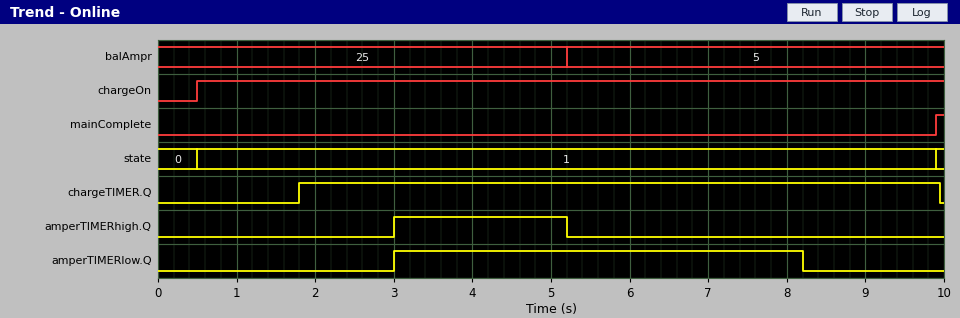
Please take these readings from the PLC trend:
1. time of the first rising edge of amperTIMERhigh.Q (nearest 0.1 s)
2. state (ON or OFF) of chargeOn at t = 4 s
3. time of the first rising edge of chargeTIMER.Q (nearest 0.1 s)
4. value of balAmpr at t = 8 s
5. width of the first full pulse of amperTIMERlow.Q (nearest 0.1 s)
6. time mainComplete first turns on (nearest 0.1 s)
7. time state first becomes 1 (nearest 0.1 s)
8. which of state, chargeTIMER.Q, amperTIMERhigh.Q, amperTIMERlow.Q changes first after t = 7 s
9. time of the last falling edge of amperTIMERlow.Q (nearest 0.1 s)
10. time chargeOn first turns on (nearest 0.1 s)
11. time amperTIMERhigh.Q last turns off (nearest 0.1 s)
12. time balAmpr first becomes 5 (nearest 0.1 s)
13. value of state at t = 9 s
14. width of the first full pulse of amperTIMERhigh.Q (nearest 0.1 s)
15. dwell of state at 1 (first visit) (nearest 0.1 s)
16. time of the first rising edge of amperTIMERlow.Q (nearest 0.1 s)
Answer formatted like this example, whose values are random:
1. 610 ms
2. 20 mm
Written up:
1. 3.0 s
2. ON
3. 1.8 s
4. 5
5. 5.2 s
6. 9.9 s
7. 0.5 s
8. amperTIMERlow.Q
9. 8.2 s
10. 0.5 s
11. 5.2 s
12. 5.2 s
13. 1
14. 2.2 s
15. 9.4 s
16. 3.0 s
